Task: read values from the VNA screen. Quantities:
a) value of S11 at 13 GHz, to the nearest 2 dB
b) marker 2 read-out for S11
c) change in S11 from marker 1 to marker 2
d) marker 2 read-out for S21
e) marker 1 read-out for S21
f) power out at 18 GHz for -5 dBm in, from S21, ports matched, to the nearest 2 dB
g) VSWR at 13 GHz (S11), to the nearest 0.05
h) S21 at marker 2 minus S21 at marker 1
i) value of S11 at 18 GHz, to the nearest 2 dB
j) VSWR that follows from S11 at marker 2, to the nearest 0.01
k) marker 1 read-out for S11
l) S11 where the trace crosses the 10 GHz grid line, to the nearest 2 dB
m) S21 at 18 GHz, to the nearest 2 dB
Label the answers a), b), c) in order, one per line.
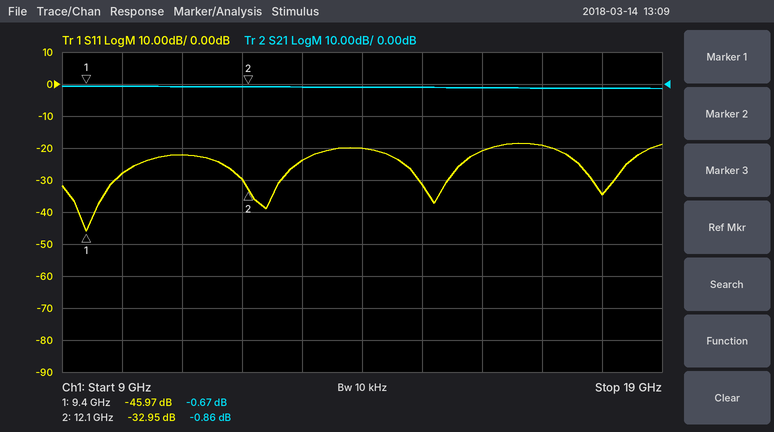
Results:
a) -24 dB
b) -32.95 dB
c) 13.02 dB
d) -0.86 dB
e) -0.67 dB
f) -6 dBm
g) 1.15
h) -0.19 dB
i) -34 dB
j) 1.05
k) -45.97 dB
l) -28 dB
m) -2 dB
